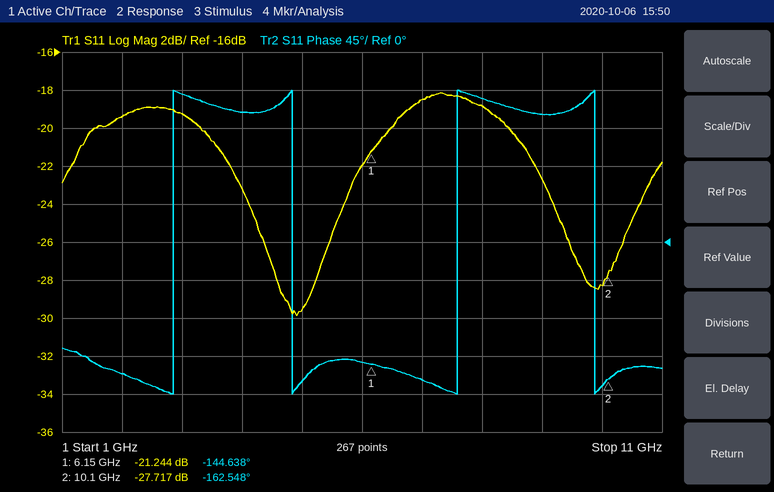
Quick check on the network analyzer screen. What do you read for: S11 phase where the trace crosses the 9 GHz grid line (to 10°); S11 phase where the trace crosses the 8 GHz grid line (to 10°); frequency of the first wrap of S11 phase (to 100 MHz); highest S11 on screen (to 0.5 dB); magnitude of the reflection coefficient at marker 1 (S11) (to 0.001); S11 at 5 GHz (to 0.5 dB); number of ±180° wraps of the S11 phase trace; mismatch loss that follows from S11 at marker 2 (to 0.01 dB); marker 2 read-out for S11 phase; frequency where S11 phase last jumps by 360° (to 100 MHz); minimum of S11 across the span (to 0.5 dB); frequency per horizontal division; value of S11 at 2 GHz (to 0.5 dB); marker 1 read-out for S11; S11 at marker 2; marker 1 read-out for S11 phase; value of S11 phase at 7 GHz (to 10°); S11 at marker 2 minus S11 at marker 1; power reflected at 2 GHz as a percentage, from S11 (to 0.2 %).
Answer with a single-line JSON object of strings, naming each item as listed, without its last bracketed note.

{"S11 phase where the trace crosses the 9 GHz grid line": "150°", "S11 phase where the trace crosses the 8 GHz grid line": "170°", "frequency of the first wrap of S11 phase": "2.9 GHz", "highest S11 on screen": "-18.0 dB", "magnitude of the reflection coefficient at marker 1 (S11)": "0.087", "S11 at 5 GHz": "-29.5 dB", "number of ±180° wraps of the S11 phase trace": "4", "mismatch loss that follows from S11 at marker 2": "0.01 dB", "marker 2 read-out for S11 phase": "-162.548°", "frequency where S11 phase last jumps by 360°": "9.9 GHz", "minimum of S11 across the span": "-30.0 dB", "frequency per horizontal division": "1 GHz", "value of S11 at 2 GHz": "-19.5 dB", "marker 1 read-out for S11": "-21.244 dB", "S11 at marker 2": "-27.717 dB", "marker 1 read-out for S11 phase": "-144.638°", "value of S11 phase at 7 GHz": "-160°", "S11 at marker 2 minus S11 at marker 1": "-6.473 dB", "power reflected at 2 GHz as a percentage, from S11": "1.2 %"}
